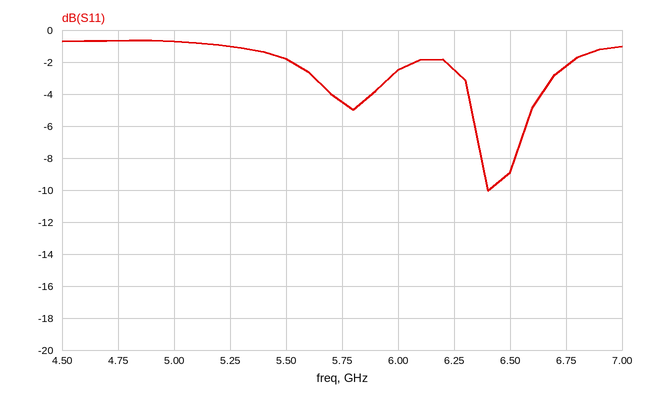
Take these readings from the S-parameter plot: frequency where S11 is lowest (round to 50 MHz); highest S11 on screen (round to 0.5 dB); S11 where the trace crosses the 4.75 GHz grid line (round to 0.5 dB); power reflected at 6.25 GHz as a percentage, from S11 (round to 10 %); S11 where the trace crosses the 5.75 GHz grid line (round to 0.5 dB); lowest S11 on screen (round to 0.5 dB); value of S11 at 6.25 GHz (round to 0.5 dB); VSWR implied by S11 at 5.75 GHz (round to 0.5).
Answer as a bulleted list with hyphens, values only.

- 6.40 GHz
- -0.5 dB
- -0.5 dB
- 60 %
- -4.5 dB
- -10.0 dB
- -2.5 dB
- 4.0
